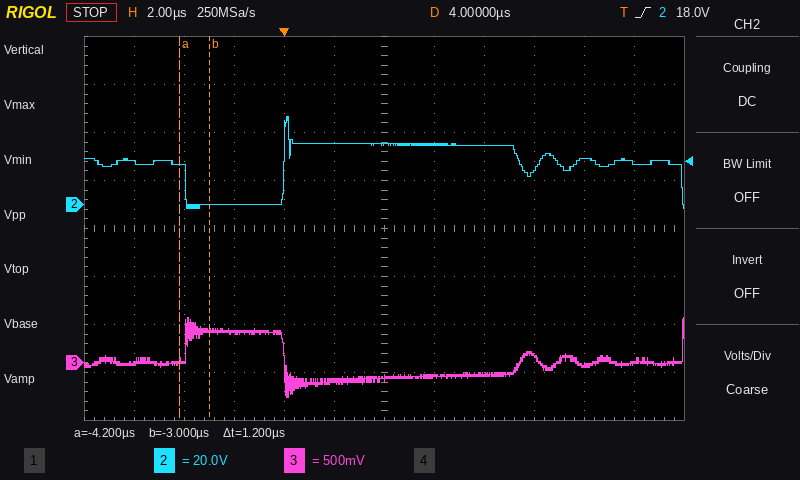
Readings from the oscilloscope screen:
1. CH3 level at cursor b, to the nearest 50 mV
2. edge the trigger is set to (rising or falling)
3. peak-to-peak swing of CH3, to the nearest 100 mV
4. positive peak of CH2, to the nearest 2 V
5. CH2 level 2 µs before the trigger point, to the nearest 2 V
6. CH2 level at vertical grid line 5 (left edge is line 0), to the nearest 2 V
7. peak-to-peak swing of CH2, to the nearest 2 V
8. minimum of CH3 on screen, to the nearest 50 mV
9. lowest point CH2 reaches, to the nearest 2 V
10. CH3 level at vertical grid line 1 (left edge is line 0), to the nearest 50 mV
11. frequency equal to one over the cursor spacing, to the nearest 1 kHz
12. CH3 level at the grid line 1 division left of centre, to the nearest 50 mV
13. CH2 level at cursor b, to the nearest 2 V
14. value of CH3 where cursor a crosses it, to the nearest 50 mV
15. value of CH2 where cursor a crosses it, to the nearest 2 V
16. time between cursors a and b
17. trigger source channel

350 mV
rising
800 mV
36 V
0 V
26 V
38 V
-350 mV
-2 V
0 mV
833 kHz
-200 mV
0 V
0 mV
16 V
1.2 µs
CH2
